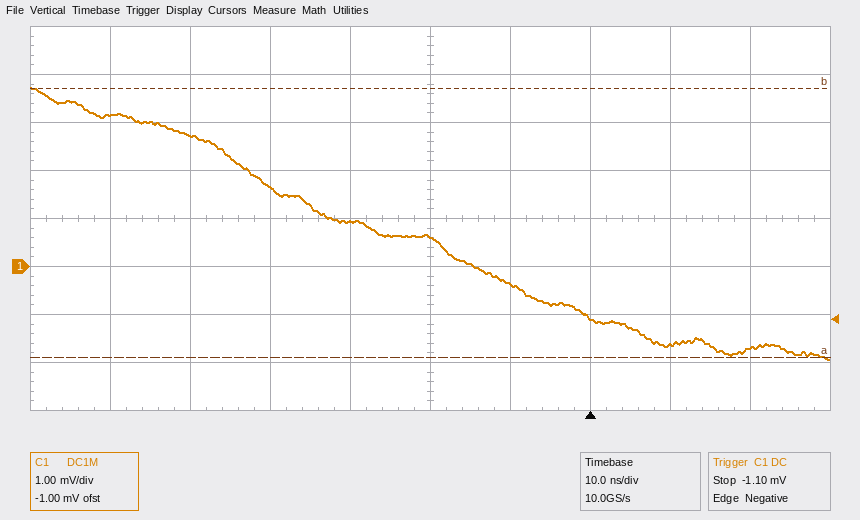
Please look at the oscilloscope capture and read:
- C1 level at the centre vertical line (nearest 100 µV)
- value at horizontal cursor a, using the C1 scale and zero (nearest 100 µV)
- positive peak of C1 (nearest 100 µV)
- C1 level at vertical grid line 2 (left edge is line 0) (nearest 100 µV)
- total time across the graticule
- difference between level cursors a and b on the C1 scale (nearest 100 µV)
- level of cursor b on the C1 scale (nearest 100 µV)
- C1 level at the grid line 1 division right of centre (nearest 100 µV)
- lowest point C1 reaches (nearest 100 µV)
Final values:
600 µV
-1.9 mV
3.7 mV
2.7 mV
100 ns
5.6 mV
3.7 mV
-400 µV
-1.9 mV
